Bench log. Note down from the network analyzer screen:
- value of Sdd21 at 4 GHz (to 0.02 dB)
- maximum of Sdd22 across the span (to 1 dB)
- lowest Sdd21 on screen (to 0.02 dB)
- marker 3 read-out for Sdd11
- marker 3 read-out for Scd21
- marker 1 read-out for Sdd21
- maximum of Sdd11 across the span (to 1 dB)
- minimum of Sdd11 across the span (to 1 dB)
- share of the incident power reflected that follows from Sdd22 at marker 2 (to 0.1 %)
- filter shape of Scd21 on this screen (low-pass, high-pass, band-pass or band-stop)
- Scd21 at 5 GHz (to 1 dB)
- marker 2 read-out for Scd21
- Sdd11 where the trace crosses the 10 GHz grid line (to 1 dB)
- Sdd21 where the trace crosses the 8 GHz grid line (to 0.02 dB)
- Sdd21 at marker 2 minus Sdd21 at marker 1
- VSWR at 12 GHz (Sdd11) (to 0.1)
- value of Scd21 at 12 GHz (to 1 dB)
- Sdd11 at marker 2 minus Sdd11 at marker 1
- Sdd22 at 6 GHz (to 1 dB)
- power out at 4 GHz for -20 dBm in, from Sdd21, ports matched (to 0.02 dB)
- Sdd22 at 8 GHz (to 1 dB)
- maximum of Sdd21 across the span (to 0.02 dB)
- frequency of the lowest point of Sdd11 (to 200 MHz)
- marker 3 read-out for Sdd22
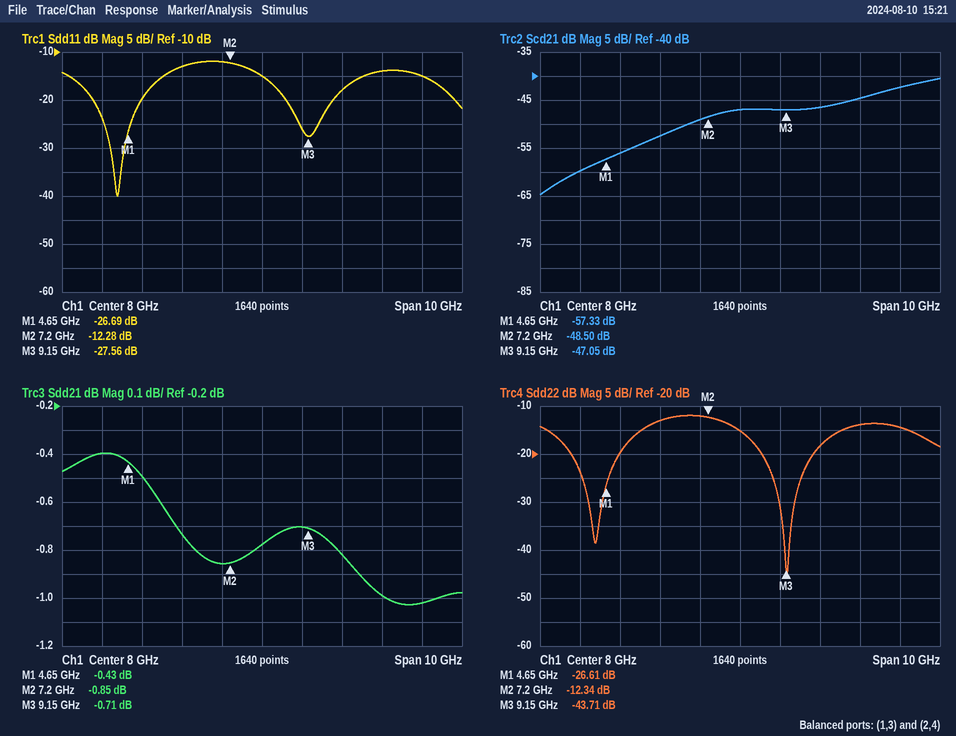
-0.40 dB
-12 dB
-1.02 dB
-27.56 dB
-47.05 dB
-0.43 dB
-12 dB
-40 dB
5.8 %
high-pass
-56 dB
-48.50 dB
-18 dB
-0.78 dB
-0.42 dB
1.4
-42 dB
14.41 dB
-13 dB
-20.40 dBm
-15 dB
-0.40 dB
4.4 GHz
-43.71 dB
